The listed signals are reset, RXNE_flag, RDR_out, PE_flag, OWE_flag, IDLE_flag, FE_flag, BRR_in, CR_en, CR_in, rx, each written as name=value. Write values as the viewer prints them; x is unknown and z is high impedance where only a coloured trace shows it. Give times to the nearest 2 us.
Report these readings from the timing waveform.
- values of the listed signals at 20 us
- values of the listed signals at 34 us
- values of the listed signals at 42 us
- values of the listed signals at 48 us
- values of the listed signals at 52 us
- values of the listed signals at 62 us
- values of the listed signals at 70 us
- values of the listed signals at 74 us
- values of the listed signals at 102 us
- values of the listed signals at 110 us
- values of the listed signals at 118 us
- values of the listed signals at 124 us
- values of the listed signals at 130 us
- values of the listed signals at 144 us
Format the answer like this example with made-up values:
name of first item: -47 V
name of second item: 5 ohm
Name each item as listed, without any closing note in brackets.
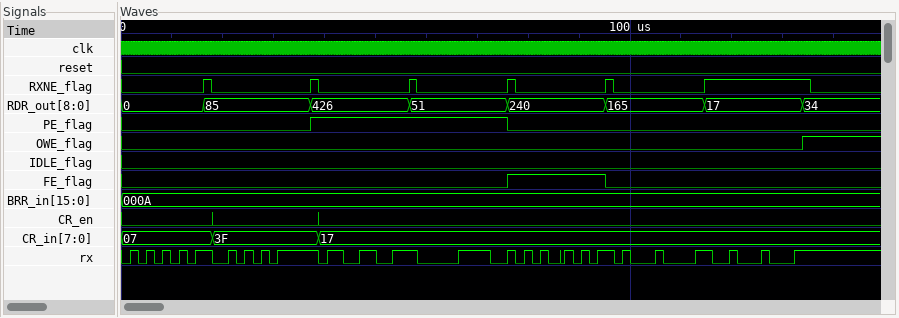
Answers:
values of the listed signals at 20 us: reset=0, RXNE_flag=0, RDR_out=85, PE_flag=0, OWE_flag=0, IDLE_flag=0, FE_flag=0, BRR_in=000A, CR_en=0, CR_in=3F, rx=0
values of the listed signals at 34 us: reset=0, RXNE_flag=0, RDR_out=85, PE_flag=0, OWE_flag=0, IDLE_flag=0, FE_flag=0, BRR_in=000A, CR_en=0, CR_in=3F, rx=1
values of the listed signals at 42 us: reset=0, RXNE_flag=0, RDR_out=426, PE_flag=1, OWE_flag=0, IDLE_flag=0, FE_flag=0, BRR_in=000A, CR_en=0, CR_in=17, rx=1
values of the listed signals at 48 us: reset=0, RXNE_flag=0, RDR_out=426, PE_flag=1, OWE_flag=0, IDLE_flag=0, FE_flag=0, BRR_in=000A, CR_en=0, CR_in=17, rx=1
values of the listed signals at 52 us: reset=0, RXNE_flag=0, RDR_out=426, PE_flag=1, OWE_flag=0, IDLE_flag=0, FE_flag=0, BRR_in=000A, CR_en=0, CR_in=17, rx=0
values of the listed signals at 62 us: reset=0, RXNE_flag=0, RDR_out=51, PE_flag=1, OWE_flag=0, IDLE_flag=0, FE_flag=0, BRR_in=000A, CR_en=0, CR_in=17, rx=0
values of the listed signals at 70 us: reset=0, RXNE_flag=0, RDR_out=51, PE_flag=1, OWE_flag=0, IDLE_flag=0, FE_flag=0, BRR_in=000A, CR_en=0, CR_in=17, rx=1
values of the listed signals at 74 us: reset=0, RXNE_flag=0, RDR_out=51, PE_flag=1, OWE_flag=0, IDLE_flag=0, FE_flag=0, BRR_in=000A, CR_en=0, CR_in=17, rx=0
values of the listed signals at 102 us: reset=0, RXNE_flag=0, RDR_out=165, PE_flag=0, OWE_flag=0, IDLE_flag=0, FE_flag=0, BRR_in=000A, CR_en=0, CR_in=17, rx=0
values of the listed signals at 110 us: reset=0, RXNE_flag=0, RDR_out=165, PE_flag=0, OWE_flag=0, IDLE_flag=0, FE_flag=0, BRR_in=000A, CR_en=0, CR_in=17, rx=0
values of the listed signals at 118 us: reset=0, RXNE_flag=1, RDR_out=17, PE_flag=0, OWE_flag=0, IDLE_flag=0, FE_flag=0, BRR_in=000A, CR_en=0, CR_in=17, rx=0
values of the listed signals at 124 us: reset=0, RXNE_flag=1, RDR_out=17, PE_flag=0, OWE_flag=0, IDLE_flag=0, FE_flag=0, BRR_in=000A, CR_en=0, CR_in=17, rx=0
values of the listed signals at 130 us: reset=0, RXNE_flag=1, RDR_out=17, PE_flag=0, OWE_flag=0, IDLE_flag=0, FE_flag=0, BRR_in=000A, CR_en=0, CR_in=17, rx=0
values of the listed signals at 144 us: reset=0, RXNE_flag=0, RDR_out=34, PE_flag=0, OWE_flag=1, IDLE_flag=0, FE_flag=0, BRR_in=000A, CR_en=0, CR_in=17, rx=1
